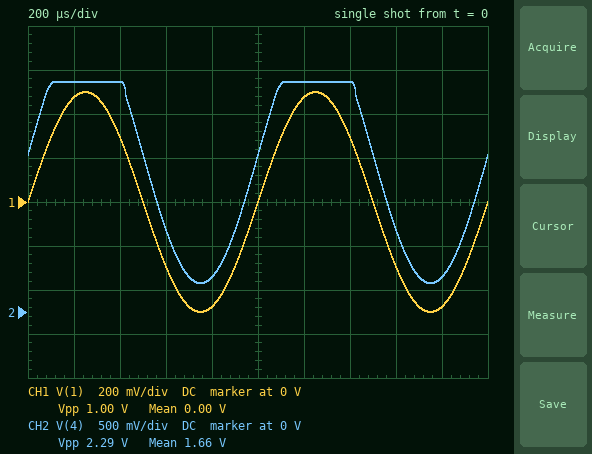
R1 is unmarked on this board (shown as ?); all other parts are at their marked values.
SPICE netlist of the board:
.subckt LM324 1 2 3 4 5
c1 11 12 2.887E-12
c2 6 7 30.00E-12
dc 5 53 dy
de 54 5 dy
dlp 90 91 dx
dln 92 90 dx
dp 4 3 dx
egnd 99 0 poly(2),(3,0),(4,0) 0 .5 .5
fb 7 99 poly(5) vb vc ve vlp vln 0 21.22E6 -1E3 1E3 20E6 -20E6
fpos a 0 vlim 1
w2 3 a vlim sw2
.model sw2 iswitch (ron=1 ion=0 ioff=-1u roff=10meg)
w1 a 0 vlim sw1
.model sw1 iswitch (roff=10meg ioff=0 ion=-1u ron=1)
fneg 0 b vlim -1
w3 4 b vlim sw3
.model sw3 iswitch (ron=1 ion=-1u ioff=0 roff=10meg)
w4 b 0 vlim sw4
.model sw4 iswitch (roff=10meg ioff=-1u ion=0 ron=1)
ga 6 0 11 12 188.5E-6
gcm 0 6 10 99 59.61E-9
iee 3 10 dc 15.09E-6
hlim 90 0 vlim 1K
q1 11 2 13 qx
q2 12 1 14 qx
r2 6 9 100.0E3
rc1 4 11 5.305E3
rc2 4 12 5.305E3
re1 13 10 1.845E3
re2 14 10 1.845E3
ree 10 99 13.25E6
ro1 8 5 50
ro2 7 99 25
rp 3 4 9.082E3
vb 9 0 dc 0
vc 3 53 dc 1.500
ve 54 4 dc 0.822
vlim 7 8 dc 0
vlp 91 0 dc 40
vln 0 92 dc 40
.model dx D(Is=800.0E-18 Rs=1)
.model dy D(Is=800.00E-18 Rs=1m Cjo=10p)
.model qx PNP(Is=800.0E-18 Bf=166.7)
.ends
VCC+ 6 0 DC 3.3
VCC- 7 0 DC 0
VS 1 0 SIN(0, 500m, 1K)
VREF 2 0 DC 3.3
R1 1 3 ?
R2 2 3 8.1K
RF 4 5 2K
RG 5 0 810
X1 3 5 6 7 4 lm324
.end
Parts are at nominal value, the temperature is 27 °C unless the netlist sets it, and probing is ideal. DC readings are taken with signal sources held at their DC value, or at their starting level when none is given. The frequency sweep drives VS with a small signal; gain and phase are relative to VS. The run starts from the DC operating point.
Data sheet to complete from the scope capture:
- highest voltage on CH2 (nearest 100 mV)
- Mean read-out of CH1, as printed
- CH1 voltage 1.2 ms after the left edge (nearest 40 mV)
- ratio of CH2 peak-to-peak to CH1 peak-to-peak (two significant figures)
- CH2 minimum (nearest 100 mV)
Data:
2.6 V
0.00 V
480 mV
2.3
300 mV
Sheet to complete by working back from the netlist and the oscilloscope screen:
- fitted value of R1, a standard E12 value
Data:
1.5 kΩ
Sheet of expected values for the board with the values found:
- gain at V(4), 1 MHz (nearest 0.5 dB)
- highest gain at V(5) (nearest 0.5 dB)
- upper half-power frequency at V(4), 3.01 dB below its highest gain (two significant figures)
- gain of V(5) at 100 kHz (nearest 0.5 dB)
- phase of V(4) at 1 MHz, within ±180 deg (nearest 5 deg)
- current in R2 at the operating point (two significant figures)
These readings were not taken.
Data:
-1.5 dB
-1.5 dB
300 kHz
-2.0 dB
-85 deg
340 µA
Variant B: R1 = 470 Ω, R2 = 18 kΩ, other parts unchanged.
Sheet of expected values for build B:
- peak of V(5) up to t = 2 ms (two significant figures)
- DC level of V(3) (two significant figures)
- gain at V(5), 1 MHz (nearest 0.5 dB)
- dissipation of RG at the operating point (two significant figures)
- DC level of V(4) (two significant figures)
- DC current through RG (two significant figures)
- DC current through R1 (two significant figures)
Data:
570 mV
84 mV
-11.0 dB
8.8 µW
290 mV
100 µA
180 µA
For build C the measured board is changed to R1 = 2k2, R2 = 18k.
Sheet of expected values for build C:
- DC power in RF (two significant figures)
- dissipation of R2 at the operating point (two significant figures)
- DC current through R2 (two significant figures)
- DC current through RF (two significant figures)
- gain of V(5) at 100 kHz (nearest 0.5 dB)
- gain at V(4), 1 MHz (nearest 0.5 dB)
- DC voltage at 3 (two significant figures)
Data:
390 µW
480 µW
160 µA
440 µA
-1.5 dB
-1.0 dB
360 mV
